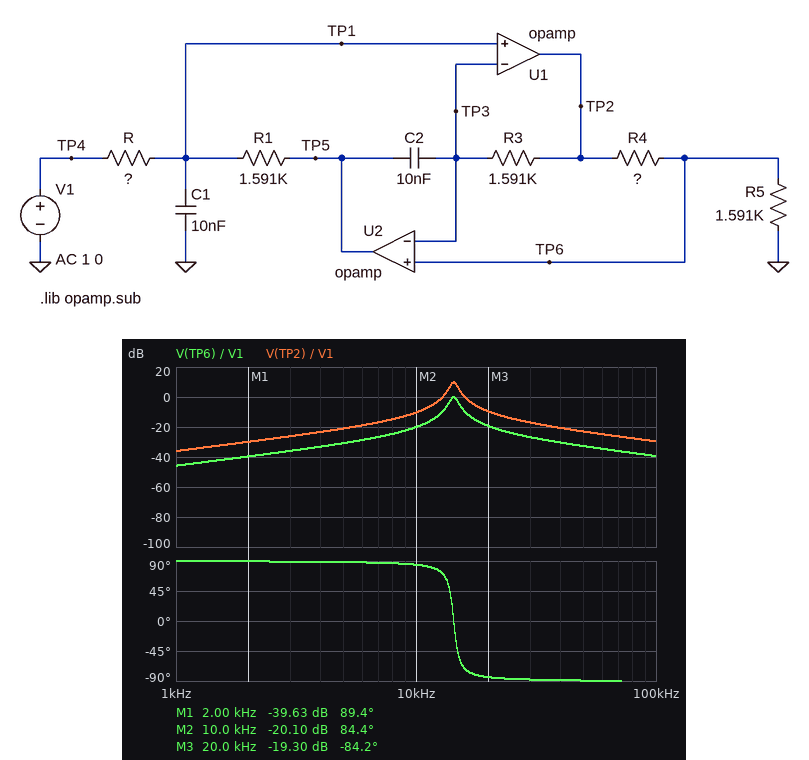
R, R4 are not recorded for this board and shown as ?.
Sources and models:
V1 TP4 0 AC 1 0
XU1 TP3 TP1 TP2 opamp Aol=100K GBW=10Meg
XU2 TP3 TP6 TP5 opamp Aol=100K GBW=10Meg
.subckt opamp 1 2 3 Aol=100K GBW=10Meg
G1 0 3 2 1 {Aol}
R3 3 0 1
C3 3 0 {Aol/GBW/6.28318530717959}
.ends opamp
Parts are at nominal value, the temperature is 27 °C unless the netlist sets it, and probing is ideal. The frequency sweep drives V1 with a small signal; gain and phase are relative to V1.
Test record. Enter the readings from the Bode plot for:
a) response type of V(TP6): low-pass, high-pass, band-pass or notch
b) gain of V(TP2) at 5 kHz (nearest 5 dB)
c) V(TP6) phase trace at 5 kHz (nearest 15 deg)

band-pass
-20 dB
90 deg
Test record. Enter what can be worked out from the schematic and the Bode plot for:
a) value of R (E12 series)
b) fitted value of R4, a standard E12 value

15 kΩ
3.3 kΩ
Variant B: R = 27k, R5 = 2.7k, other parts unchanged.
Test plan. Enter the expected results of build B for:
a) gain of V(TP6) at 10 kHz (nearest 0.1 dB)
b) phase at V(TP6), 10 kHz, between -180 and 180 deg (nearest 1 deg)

-11.7 dB
75 deg
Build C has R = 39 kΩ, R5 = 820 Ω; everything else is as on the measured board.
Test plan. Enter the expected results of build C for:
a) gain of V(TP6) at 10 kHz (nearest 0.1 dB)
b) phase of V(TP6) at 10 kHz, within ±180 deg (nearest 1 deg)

-37.4 dB
89 deg
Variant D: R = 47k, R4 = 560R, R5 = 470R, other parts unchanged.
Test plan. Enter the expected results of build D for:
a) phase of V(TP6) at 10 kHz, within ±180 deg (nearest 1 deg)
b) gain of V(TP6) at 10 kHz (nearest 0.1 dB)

80 deg
-15.0 dB
